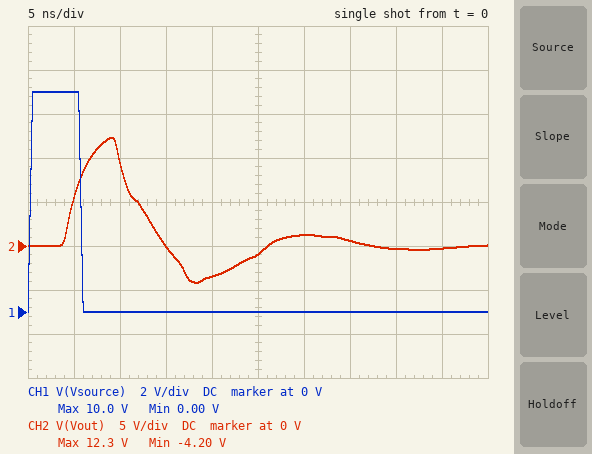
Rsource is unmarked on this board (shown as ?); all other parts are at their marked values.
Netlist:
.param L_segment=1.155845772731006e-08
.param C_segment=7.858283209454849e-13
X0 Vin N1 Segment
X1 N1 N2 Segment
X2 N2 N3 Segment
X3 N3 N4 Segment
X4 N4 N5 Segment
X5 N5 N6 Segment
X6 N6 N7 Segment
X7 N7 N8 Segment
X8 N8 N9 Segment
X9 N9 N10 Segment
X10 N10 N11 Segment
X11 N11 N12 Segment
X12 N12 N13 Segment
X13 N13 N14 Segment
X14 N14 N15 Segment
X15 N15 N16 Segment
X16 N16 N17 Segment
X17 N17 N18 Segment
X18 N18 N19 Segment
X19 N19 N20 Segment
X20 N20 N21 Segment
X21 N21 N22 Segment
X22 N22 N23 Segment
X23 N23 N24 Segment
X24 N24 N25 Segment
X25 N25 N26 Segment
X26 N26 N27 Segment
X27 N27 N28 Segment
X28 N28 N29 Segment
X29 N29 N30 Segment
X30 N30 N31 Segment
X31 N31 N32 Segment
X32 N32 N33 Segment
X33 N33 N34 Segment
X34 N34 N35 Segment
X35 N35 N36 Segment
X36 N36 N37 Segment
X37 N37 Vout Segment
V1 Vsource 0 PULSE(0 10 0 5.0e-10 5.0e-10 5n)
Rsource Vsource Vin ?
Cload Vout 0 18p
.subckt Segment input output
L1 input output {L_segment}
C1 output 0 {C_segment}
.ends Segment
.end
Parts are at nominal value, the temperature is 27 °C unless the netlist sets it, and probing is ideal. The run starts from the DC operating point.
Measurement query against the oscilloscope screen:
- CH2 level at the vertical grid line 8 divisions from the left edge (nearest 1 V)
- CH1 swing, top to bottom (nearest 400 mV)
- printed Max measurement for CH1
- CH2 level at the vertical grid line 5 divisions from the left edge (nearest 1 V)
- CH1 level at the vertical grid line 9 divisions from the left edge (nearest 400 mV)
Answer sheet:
0 V
10.0 V
10.0 V
-1 V
0 V
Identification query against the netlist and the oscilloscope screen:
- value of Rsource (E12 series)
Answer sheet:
56 Ω
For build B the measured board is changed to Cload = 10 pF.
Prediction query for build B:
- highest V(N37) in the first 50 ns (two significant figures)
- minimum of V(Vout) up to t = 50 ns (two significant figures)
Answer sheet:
13 V
-5.7 V
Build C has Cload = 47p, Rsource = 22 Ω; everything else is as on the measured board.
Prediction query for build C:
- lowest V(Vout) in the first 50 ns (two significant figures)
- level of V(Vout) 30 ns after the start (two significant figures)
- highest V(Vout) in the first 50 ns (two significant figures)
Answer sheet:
-6.3 V
-4.1 V
10 V
